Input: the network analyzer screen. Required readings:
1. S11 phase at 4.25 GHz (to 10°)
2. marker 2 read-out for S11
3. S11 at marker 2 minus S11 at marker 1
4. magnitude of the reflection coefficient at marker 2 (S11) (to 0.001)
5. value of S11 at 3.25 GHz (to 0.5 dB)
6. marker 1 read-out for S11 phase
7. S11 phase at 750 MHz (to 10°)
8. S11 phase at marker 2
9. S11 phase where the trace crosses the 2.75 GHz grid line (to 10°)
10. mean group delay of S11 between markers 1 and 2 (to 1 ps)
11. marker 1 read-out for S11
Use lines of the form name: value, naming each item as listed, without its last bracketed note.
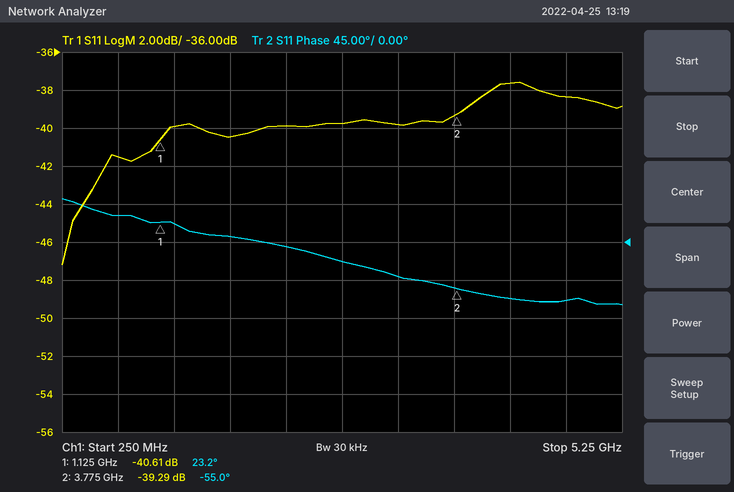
S11 phase at 4.25 GHz: -70°
marker 2 read-out for S11: -39.29 dB
S11 at marker 2 minus S11 at marker 1: 1.32 dB
magnitude of the reflection coefficient at marker 2 (S11): 0.011
value of S11 at 3.25 GHz: -40.0 dB
marker 1 read-out for S11 phase: 23.2°
S11 phase at 750 MHz: 30°
S11 phase at marker 2: -55.0°
S11 phase where the trace crosses the 2.75 GHz grid line: -20°
mean group delay of S11 between markers 1 and 2: 82 ps
marker 1 read-out for S11: -40.61 dB
